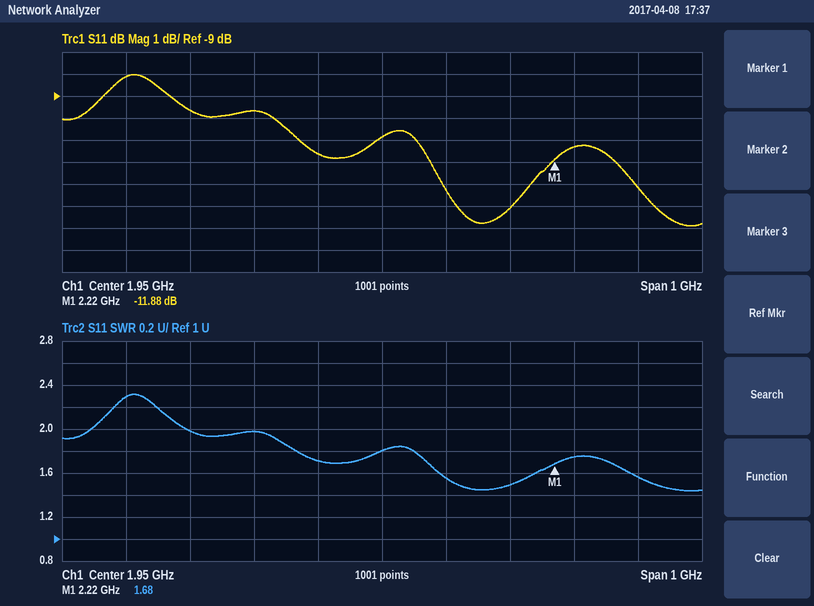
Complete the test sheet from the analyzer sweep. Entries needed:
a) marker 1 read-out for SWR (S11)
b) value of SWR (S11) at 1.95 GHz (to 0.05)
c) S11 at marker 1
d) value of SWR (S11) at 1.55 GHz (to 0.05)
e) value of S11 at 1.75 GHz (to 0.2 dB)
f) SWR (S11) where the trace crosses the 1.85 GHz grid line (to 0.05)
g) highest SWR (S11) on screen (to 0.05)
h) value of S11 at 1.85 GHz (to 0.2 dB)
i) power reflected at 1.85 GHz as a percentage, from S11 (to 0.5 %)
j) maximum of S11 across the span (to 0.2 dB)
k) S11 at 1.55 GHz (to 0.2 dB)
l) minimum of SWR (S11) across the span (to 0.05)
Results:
1.68
1.80
-11.88 dB
2.30
-9.6 dB
1.70
2.30
-11.6 dB
7.0 %
-8.0 dB
-8.2 dB
1.45
